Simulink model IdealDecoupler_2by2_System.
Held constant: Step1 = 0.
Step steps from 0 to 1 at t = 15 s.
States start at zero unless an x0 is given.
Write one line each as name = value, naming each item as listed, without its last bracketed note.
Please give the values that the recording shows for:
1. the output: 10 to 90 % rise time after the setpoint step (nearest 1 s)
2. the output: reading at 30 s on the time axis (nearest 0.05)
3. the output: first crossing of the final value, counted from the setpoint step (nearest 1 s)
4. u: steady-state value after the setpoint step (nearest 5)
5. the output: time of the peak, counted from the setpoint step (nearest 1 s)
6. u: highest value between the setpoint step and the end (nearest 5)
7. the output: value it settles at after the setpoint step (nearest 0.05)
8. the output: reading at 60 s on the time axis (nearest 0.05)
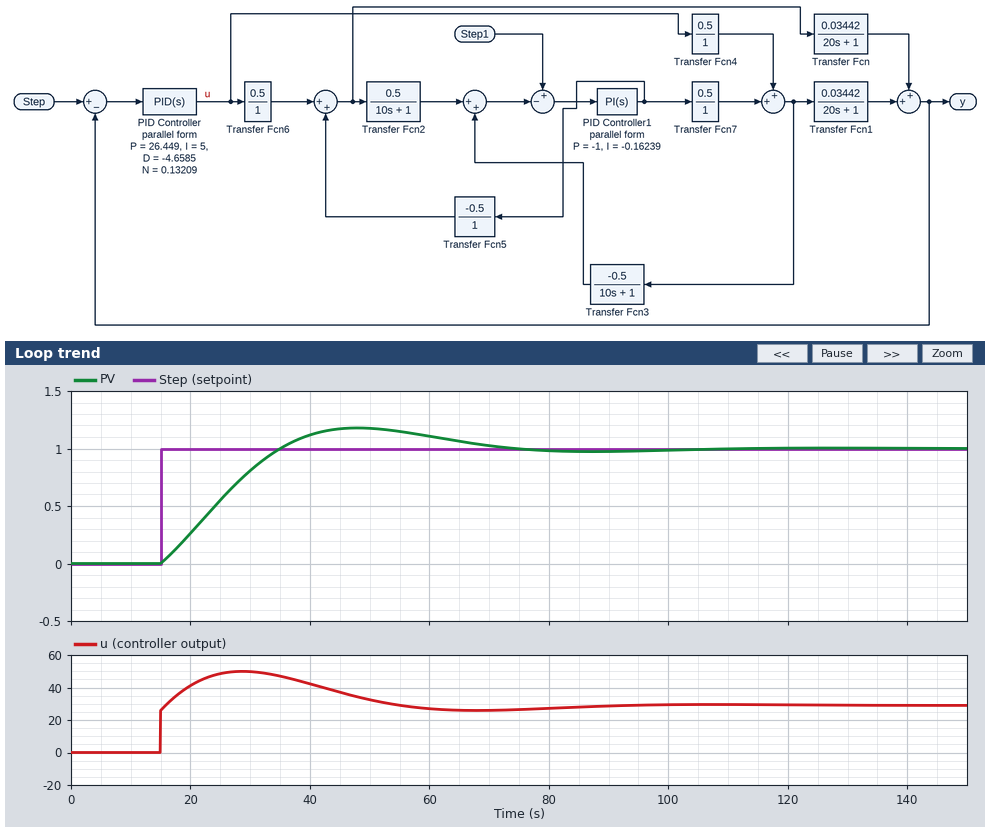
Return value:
the output: 10 to 90 % rise time after the setpoint step = 15 s
the output: reading at 30 s on the time axis = 0.80
the output: first crossing of the final value, counted from the setpoint step = 20 s
u: steady-state value after the setpoint step = 30
the output: time of the peak, counted from the setpoint step = 33 s
u: highest value between the setpoint step and the end = 50
the output: value it settles at after the setpoint step = 1.00
the output: reading at 60 s on the time axis = 1.10
